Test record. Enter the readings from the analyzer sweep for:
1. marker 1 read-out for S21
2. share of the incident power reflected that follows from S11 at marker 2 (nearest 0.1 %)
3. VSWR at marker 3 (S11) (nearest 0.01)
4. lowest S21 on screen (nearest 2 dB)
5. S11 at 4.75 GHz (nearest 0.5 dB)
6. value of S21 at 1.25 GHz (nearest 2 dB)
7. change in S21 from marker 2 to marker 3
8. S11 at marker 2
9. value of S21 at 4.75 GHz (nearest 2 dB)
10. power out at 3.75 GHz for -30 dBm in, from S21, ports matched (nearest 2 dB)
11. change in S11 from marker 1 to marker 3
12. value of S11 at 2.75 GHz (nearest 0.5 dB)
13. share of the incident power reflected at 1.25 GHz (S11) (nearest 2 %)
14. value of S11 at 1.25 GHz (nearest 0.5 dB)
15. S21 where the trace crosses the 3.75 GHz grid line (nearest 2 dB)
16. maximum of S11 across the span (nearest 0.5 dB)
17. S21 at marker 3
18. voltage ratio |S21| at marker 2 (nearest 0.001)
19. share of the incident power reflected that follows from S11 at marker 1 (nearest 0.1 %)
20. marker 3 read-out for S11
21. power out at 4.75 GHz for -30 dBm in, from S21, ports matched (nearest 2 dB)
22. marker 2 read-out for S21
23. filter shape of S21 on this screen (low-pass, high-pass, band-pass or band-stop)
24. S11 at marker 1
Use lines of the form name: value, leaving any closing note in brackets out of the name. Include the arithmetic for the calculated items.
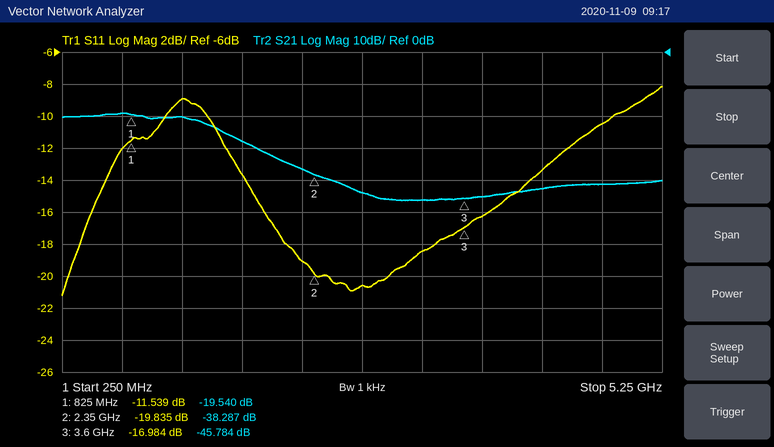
marker 1 read-out for S21: -19.540 dB
share of the incident power reflected that follows from S11 at marker 2: 10^(-19.835/10) ≈ 1.0 %
VSWR at marker 3 (S11): (1 + 0.1415)/(1 − 0.1415) ≈ 1.33
lowest S21 on screen: -46 dB
S11 at 4.75 GHz: -10.5 dB
value of S21 at 1.25 GHz: -20 dB
change in S21 from marker 2 to marker 3: -45.784 − (-38.287) = -7.497 dB
S11 at marker 2: -19.835 dB
value of S21 at 4.75 GHz: -42 dB
power out at 3.75 GHz for -30 dBm in, from S21, ports matched: -30 dBm + (-46 dB) = -76 dBm
change in S11 from marker 1 to marker 3: -16.984 − (-11.539) = -5.445 dB
value of S11 at 2.75 GHz: -20.5 dB
share of the incident power reflected at 1.25 GHz (S11): 10^(-9/10) ≈ 12.6 %, so 12 % to the nearest 2 %
value of S11 at 1.25 GHz: -9.0 dB
S21 where the trace crosses the 3.75 GHz grid line: -46 dB
maximum of S11 across the span: -8.0 dB
S21 at marker 3: -45.784 dB
voltage ratio |S21| at marker 2: 10^(-38.287/20) ≈ 0.012
share of the incident power reflected that follows from S11 at marker 1: 10^(-11.539/10) ≈ 7.0 %
marker 3 read-out for S11: -16.984 dB
power out at 4.75 GHz for -30 dBm in, from S21, ports matched: -30 dBm + (-42 dB) = -72 dBm
marker 2 read-out for S21: -38.287 dB
filter shape of S21 on this screen: low-pass
S11 at marker 1: -11.539 dB
